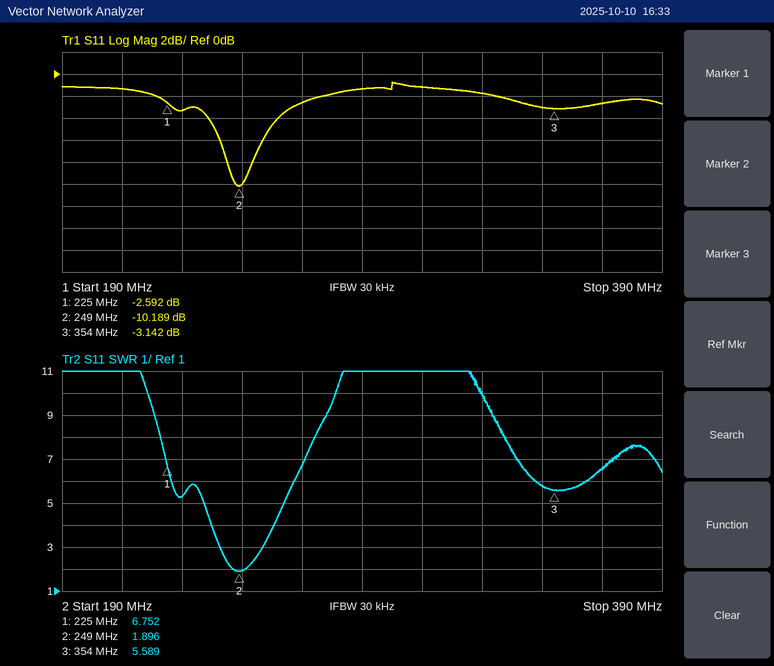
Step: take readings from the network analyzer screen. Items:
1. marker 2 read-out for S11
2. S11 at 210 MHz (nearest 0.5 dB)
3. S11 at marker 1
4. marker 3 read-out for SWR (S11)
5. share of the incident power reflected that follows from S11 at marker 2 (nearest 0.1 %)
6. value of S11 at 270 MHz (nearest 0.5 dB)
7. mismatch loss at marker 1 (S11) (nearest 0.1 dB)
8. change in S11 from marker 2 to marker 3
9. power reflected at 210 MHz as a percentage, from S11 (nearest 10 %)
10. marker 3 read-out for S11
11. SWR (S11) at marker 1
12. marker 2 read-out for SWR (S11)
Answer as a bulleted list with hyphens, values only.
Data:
- -10.189 dB
- -1.5 dB
- -2.592 dB
- 5.589
- 9.6 %
- -2.5 dB
- 3.5 dB
- 7.047 dB
- 70 %
- -3.142 dB
- 6.752
- 1.896
